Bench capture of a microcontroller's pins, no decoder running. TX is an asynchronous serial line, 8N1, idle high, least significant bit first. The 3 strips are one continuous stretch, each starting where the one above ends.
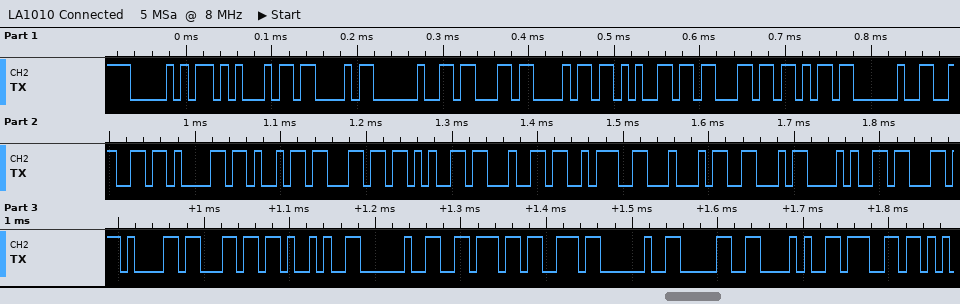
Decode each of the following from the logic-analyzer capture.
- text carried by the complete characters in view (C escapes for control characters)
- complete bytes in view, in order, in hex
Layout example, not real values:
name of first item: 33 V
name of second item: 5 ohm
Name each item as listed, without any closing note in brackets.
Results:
text carried by the complete characters in view: "PEC check failed:DF(cal) vs 0(g"
complete bytes in view, in order, in hex: 50 45 43 20 63 68 65 63 6B 20 66 61 69 6C 65 64 3A 44 46 28 63 61 6C 29 20 76 73 20 30 28 67
